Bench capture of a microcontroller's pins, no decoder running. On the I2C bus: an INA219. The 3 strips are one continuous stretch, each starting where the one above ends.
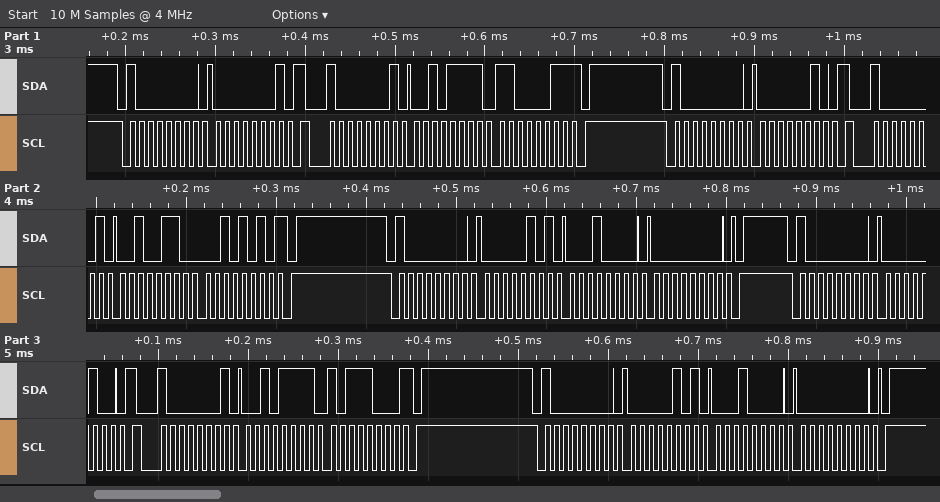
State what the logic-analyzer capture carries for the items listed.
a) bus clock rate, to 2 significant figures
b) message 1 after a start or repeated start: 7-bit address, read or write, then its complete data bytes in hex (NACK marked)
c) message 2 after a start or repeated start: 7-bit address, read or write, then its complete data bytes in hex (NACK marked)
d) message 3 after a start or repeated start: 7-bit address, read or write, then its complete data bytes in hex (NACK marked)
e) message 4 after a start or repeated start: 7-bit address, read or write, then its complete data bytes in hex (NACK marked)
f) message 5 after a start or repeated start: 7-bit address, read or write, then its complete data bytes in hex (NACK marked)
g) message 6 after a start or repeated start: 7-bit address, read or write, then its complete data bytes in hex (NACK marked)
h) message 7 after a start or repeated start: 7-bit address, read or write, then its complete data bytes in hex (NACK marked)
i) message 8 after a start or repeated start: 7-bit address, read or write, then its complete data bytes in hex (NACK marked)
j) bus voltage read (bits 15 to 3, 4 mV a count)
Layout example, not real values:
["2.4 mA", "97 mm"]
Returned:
["100 kHz", "0x40 write: 01", "0x40 read: 2F C3 NACK", "0x40 write: 02", "0x40 read: 26 2A NACK", "0x40 write: 05 10 00", "0x40 write: 04", "0x40 read: 2F B8 NACK", "0x40 write: 05 10 00", "4.884 V"]
